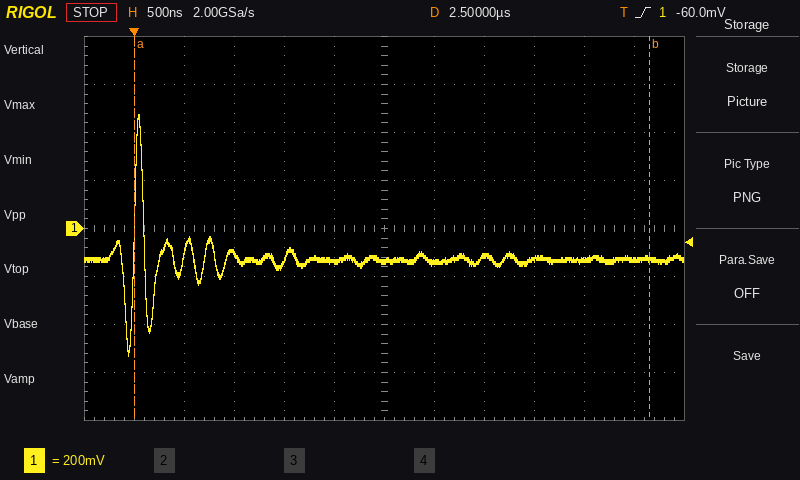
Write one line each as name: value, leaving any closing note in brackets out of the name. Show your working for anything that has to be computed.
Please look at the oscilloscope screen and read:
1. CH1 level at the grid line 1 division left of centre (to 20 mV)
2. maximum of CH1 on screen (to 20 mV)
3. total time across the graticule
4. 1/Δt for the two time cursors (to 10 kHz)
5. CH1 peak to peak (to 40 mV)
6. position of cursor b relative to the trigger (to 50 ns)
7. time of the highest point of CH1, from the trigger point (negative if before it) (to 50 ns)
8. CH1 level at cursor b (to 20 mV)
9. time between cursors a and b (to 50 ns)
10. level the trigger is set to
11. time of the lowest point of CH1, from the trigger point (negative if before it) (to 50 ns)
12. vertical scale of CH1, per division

CH1 level at the grid line 1 division left of centre: -140 mV
maximum of CH1 on screen: 480 mV
total time across the graticule: 6 µs
1/Δt for the two time cursors: 1 / 5.15 µs ≈ 190 kHz
CH1 peak to peak: 1.00 V
position of cursor b relative to the trigger: +5.15 µs
time of the highest point of CH1, from the trigger point (negative if before it): +50 ns
CH1 level at cursor b: -120 mV
time between cursors a and b: 5.15 µs
level the trigger is set to: -60.0 mV
time of the lowest point of CH1, from the trigger point (negative if before it): -50 ns
vertical scale of CH1, per division: 200 mV
